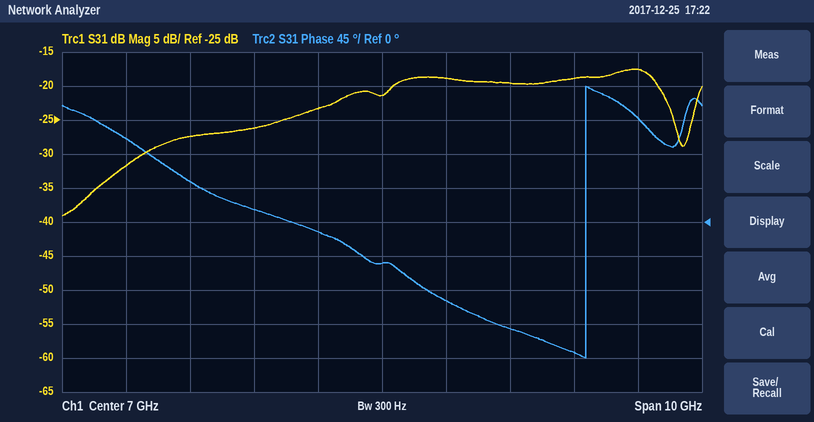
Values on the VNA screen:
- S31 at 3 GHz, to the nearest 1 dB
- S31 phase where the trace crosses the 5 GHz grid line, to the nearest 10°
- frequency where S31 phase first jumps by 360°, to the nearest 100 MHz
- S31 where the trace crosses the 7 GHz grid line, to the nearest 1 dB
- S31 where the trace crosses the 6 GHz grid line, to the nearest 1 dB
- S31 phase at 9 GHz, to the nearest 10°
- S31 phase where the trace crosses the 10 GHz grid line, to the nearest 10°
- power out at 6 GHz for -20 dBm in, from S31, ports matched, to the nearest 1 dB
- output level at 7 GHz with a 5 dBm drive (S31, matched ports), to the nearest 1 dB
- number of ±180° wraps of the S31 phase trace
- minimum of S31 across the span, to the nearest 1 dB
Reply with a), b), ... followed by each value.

a) -32 dB
b) 20°
c) 10.2 GHz
d) -21 dB
e) -23 dB
f) -140°
g) -170°
h) -43 dBm
i) -16 dBm
j) 1
k) -39 dB
